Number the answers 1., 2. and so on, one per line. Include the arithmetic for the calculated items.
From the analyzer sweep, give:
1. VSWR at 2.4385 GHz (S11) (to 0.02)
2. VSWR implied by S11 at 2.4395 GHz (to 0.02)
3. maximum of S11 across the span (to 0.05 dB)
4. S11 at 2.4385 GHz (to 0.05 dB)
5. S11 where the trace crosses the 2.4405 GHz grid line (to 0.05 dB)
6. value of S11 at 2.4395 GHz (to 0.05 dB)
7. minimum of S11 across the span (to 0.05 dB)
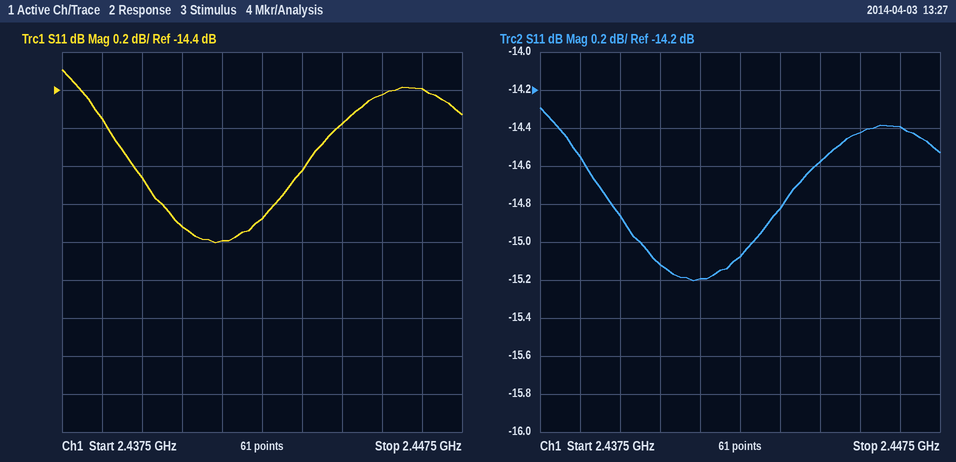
1. |Γ| = 10^(-14.55/20) = 0.1873; VSWR = (1 + 0.1873)/(1 − 0.1873) ≈ 1.46
2. |Γ| = 10^(-14.85/20) = 0.1809; VSWR = (1 + 0.1809)/(1 − 0.1809) ≈ 1.44
3. -14.30 dB
4. -14.55 dB
5. -15.10 dB
6. -14.85 dB
7. -15.20 dB
